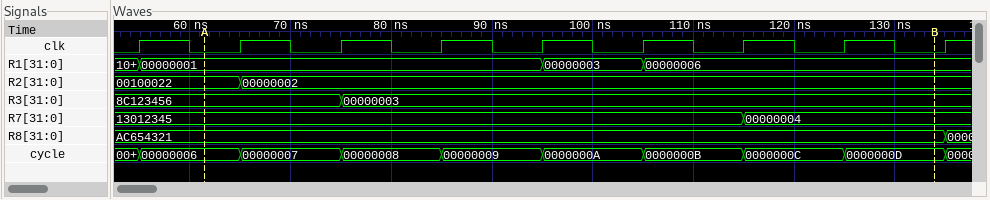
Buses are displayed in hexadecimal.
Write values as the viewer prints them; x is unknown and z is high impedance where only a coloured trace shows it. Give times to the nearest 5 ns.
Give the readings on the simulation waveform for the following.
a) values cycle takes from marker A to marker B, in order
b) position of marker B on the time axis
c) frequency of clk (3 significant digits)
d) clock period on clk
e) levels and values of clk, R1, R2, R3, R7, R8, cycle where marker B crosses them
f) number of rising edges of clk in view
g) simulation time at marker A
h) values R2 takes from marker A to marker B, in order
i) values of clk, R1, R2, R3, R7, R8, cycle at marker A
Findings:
00000006, 00000007, 00000008, 00000009, 0000000A, 0000000B, 0000000C, 0000000D
135 ns
100 MHz
10 ns
clk=0, R1=00000006, R2=00000002, R3=00000003, R7=00000004, R8=AC654321, cycle=0000000D
9
60 ns
00100022, 00000002
clk=0, R1=00000001, R2=00100022, R3=8C123456, R7=13012345, R8=AC654321, cycle=00000006
